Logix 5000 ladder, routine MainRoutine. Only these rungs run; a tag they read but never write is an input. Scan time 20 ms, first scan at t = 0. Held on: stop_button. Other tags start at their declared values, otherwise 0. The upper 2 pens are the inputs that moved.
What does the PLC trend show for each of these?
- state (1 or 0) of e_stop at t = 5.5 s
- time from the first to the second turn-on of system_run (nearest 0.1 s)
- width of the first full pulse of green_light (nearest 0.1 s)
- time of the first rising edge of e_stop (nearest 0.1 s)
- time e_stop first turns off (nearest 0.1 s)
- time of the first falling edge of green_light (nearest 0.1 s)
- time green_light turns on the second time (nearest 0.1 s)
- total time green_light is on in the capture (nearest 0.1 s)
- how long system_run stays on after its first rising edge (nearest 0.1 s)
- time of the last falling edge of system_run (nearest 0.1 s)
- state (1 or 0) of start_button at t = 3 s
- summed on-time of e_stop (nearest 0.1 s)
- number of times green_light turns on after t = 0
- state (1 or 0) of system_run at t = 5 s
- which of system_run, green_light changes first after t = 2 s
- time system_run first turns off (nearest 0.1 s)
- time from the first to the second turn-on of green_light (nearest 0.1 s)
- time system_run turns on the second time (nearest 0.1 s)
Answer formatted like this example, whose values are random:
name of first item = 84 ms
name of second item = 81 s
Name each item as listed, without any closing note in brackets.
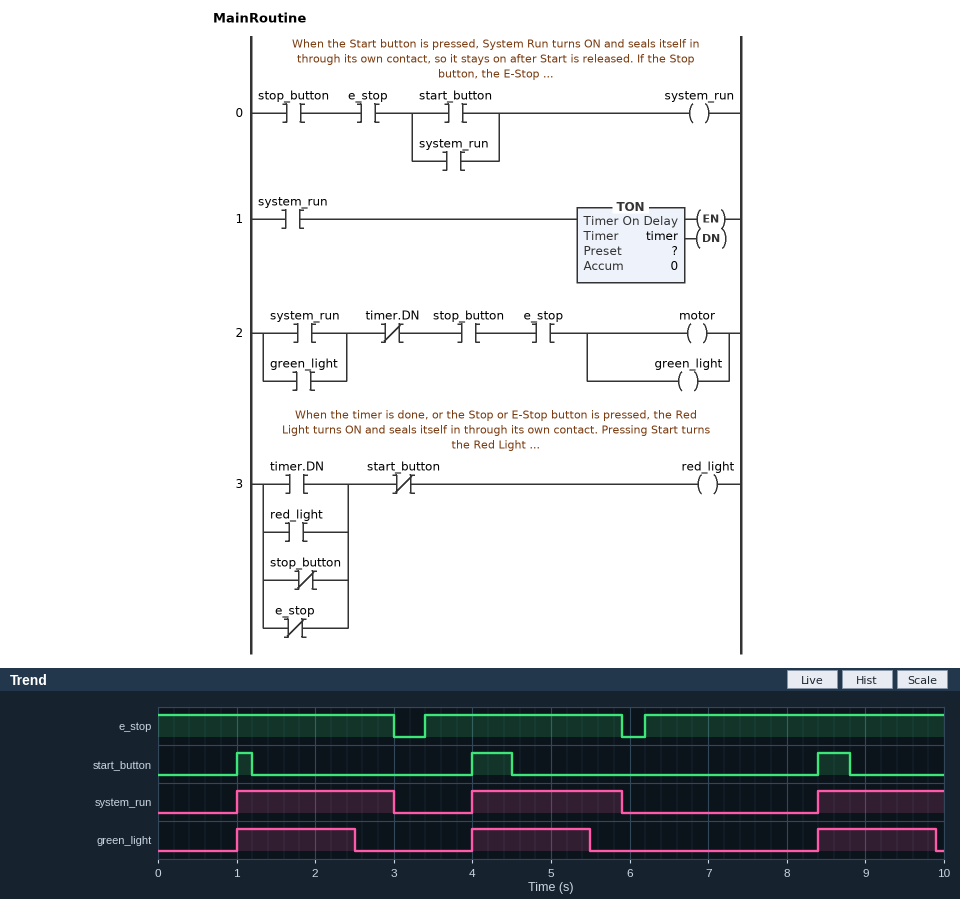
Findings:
state (1 or 0) of e_stop at t = 5.5 s = 1
time from the first to the second turn-on of system_run = 3.0 s
width of the first full pulse of green_light = 1.5 s
time of the first rising edge of e_stop = 3.4 s
time e_stop first turns off = 3.0 s
time of the first falling edge of green_light = 2.5 s
time green_light turns on the second time = 4.0 s
total time green_light is on in the capture = 4.5 s
how long system_run stays on after its first rising edge = 2.0 s
time of the last falling edge of system_run = 5.9 s
state (1 or 0) of start_button at t = 3 s = 0
summed on-time of e_stop = 9.3 s
number of times green_light turns on after t = 0 = 3
state (1 or 0) of system_run at t = 5 s = 1
which of system_run, green_light changes first after t = 2 s = green_light
time system_run first turns off = 3.0 s
time from the first to the second turn-on of green_light = 3.0 s
time system_run turns on the second time = 4.0 s
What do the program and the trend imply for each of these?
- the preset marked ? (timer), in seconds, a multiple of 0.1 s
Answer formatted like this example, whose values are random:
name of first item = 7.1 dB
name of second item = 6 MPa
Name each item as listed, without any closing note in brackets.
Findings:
the preset marked ? (timer), in seconds, a multiple of 0.1 s = 1.5 s
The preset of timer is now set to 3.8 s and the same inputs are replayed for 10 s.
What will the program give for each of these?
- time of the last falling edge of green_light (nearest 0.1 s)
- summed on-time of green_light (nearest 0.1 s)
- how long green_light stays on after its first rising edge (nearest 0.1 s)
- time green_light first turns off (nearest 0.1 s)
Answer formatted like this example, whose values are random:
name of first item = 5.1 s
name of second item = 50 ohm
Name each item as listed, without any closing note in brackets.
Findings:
time of the last falling edge of green_light = 5.9 s
summed on-time of green_light = 5.5 s
how long green_light stays on after its first rising edge = 2.0 s
time green_light first turns off = 3.0 s
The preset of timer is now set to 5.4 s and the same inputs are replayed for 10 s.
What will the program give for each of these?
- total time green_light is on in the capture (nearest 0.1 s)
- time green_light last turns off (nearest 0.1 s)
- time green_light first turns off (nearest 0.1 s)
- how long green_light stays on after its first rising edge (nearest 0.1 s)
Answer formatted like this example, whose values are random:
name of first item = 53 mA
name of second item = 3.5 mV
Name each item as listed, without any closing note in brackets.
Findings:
total time green_light is on in the capture = 5.5 s
time green_light last turns off = 5.9 s
time green_light first turns off = 3.0 s
how long green_light stays on after its first rising edge = 2.0 s
